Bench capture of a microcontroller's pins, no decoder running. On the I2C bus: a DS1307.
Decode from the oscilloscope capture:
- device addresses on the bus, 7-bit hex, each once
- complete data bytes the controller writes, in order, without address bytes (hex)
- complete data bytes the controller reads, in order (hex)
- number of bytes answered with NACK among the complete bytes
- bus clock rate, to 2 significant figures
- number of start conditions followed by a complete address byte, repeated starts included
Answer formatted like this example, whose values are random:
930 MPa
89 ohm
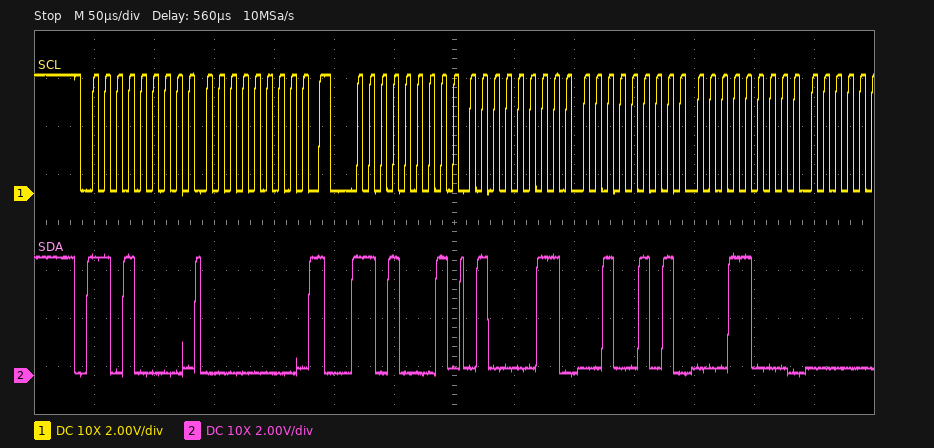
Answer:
0x68
00
43 25 18
0
100 kHz
2
